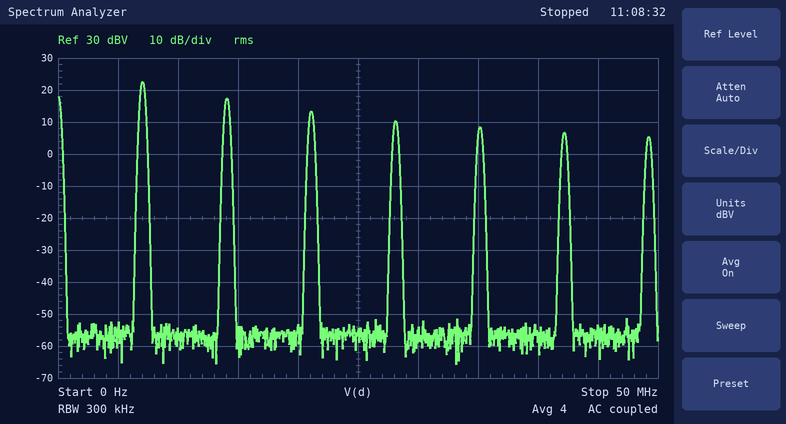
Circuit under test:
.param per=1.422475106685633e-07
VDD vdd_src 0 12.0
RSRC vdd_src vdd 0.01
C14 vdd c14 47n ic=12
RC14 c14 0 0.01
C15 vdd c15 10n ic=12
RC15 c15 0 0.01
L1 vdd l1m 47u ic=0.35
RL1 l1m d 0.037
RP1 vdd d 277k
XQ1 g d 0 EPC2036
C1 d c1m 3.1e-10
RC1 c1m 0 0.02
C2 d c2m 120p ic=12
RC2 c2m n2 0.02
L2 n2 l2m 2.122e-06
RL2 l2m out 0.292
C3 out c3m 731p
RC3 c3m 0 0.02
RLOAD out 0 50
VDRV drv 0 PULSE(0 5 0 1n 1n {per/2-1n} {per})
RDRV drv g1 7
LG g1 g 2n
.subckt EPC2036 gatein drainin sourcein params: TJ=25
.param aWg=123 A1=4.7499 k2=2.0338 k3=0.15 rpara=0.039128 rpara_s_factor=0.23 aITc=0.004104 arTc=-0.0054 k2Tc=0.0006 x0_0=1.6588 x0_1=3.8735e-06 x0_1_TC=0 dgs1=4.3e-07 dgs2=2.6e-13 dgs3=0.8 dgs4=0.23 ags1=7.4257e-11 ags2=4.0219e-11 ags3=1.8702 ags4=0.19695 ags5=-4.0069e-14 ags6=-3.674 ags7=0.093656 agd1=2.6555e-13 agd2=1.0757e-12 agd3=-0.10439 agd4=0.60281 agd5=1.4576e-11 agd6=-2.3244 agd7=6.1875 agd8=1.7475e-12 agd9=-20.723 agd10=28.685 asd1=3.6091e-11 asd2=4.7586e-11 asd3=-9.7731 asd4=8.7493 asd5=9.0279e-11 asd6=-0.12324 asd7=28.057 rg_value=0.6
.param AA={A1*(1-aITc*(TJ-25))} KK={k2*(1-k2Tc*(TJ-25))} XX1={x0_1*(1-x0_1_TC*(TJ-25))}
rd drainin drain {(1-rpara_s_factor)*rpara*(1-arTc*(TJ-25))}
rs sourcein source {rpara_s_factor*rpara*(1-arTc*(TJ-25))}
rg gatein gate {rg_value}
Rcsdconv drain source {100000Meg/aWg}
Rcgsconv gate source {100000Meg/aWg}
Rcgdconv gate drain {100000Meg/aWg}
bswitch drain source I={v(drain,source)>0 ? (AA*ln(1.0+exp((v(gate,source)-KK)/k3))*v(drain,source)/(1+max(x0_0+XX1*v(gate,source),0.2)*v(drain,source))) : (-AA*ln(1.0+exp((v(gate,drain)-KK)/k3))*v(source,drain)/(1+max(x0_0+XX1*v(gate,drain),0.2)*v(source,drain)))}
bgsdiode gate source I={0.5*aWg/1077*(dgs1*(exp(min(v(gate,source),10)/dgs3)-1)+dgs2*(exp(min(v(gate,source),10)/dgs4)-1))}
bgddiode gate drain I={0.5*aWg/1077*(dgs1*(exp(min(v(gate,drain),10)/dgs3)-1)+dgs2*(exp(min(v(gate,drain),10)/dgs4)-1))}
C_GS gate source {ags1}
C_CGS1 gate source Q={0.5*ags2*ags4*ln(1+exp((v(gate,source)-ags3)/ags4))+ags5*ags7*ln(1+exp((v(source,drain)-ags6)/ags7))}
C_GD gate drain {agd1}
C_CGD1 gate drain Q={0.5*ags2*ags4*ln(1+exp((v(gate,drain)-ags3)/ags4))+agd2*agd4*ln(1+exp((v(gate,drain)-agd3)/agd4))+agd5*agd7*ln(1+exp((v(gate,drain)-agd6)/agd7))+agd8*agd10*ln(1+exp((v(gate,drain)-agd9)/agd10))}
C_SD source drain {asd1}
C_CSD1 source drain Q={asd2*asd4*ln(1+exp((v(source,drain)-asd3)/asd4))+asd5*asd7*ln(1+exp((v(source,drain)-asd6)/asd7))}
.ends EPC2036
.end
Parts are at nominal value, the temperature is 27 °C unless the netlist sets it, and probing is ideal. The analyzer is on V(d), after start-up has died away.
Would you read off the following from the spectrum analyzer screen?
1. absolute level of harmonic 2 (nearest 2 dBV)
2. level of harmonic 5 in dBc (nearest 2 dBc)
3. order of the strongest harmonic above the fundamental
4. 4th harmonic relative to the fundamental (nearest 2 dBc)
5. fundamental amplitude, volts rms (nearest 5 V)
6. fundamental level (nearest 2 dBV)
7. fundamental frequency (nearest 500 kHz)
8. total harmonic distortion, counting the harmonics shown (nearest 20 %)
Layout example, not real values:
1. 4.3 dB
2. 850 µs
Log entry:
1. 18 dBV
2. -14 dBc
3. 2
4. -12 dBc
5. 15 V
6. 22 dBV
7. 7.0 MHz
8. 80 %
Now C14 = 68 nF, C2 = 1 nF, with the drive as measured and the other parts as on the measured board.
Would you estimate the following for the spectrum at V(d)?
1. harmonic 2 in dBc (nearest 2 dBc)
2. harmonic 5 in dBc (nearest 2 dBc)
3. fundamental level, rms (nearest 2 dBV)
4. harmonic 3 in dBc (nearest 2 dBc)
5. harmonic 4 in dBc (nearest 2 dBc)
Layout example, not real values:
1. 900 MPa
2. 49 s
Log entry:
1. -10 dBc
2. -24 dBc
3. 22 dBV
4. -20 dBc
5. -20 dBc
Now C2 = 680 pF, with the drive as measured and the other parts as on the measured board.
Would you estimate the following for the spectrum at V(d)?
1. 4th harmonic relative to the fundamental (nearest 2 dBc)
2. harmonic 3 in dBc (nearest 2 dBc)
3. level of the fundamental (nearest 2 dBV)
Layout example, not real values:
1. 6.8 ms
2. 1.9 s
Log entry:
1. -22 dBc
2. -24 dBc
3. 22 dBV
